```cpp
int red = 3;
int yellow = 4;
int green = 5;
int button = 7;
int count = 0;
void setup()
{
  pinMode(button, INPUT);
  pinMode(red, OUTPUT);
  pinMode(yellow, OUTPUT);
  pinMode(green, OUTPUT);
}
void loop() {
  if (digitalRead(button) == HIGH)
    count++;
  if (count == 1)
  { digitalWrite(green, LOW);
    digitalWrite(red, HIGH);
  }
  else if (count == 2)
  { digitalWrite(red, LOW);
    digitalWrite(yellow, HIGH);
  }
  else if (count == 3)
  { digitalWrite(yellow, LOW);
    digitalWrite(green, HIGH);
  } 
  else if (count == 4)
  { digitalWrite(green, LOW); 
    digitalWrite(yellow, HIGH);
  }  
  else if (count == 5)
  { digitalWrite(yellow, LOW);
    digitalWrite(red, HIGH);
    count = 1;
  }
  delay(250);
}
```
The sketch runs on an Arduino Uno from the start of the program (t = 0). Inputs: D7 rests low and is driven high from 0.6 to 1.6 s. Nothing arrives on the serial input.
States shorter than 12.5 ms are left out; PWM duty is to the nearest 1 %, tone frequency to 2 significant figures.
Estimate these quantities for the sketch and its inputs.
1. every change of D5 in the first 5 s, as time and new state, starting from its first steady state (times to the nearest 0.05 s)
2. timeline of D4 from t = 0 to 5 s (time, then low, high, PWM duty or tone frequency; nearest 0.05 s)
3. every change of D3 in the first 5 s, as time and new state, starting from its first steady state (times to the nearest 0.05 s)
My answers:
0 s low; 1.25 s high; 1.5 s low
0 s low; 1 s high; 1.25 s low; 1.5 s high
0 s low; 0.75 s high; 1 s low
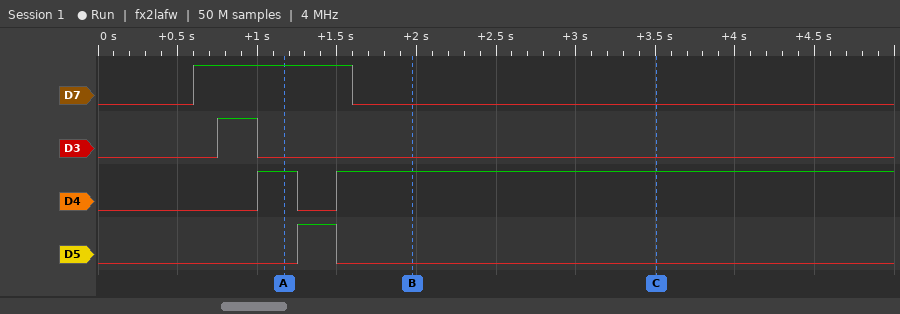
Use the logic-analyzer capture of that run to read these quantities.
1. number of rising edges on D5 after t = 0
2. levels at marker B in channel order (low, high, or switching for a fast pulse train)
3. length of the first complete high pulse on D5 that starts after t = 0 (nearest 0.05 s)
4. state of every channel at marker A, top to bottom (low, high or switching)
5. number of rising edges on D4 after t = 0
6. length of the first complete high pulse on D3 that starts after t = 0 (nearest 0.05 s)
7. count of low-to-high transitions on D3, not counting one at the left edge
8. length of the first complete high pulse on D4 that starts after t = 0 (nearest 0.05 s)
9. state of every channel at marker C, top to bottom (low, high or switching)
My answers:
1
D7 low, D3 low, D4 high, D5 low
0.25 s
D7 high, D3 low, D4 high, D5 low
2
0.25 s
1
0.25 s
D7 low, D3 low, D4 high, D5 low
